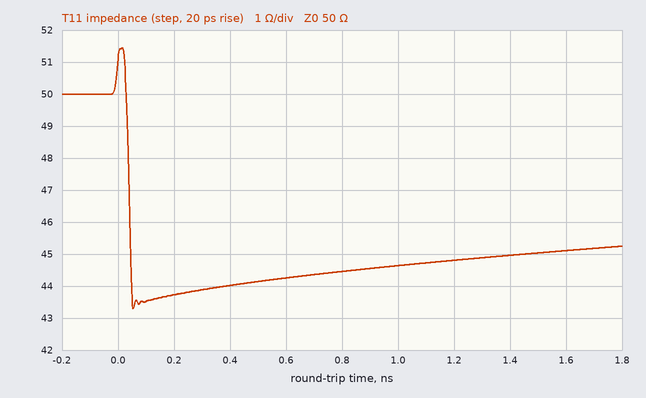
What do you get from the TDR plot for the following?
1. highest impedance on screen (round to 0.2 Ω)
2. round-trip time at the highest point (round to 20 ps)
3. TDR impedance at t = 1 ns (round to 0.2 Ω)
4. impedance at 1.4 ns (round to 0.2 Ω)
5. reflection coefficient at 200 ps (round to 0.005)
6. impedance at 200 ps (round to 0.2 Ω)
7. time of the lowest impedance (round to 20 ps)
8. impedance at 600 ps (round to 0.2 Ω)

51.4 Ω
20 ps
44.6 Ω
45.0 Ω
-0.065
43.8 Ω
60 ps
44.2 Ω
